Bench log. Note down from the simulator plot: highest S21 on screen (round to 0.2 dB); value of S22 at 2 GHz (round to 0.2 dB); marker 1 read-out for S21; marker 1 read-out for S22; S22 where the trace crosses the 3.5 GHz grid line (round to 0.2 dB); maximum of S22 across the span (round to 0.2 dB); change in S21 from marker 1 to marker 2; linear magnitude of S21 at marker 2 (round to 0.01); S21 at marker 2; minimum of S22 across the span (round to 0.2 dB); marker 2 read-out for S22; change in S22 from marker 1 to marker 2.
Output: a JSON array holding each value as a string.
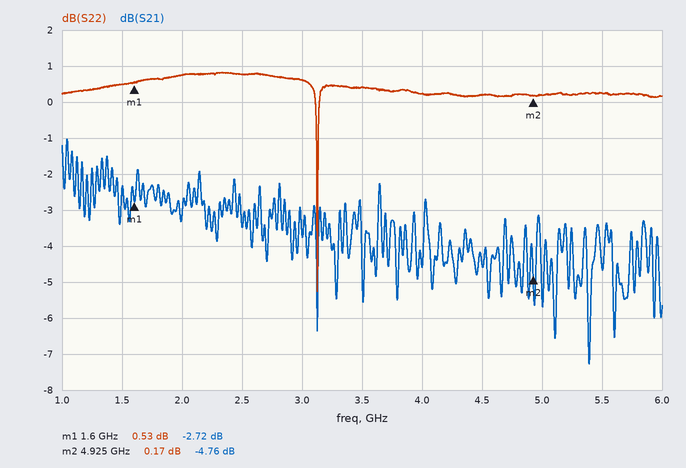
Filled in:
["-1.0 dB", "0.8 dB", "-2.72 dB", "0.53 dB", "0.4 dB", "0.8 dB", "-2.04 dB", "0.58", "-4.76 dB", "-5.2 dB", "0.17 dB", "-0.36 dB"]
